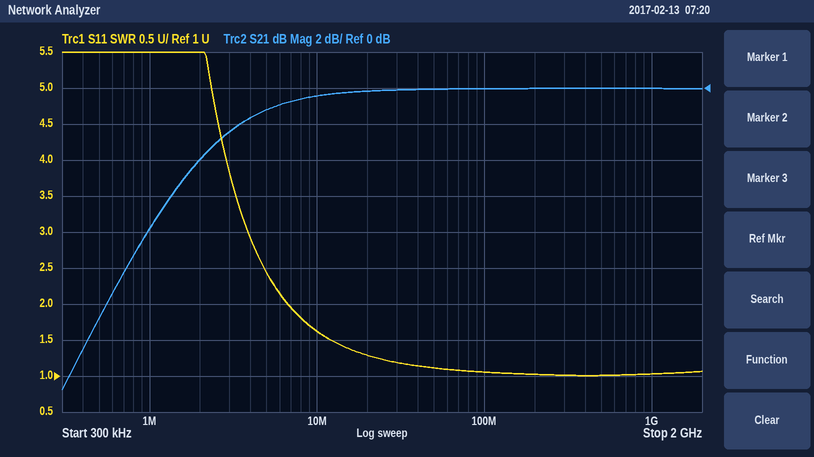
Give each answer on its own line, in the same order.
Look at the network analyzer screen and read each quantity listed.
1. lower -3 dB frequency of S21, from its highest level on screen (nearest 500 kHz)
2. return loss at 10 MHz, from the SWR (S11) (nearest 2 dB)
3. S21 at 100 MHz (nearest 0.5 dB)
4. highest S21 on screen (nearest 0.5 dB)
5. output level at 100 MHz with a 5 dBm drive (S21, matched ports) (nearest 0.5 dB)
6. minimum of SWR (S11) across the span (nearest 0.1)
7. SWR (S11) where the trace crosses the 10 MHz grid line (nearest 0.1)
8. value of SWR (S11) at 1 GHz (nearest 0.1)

2.5 MHz
12 dB
0.0 dB
0.0 dB
5.0 dBm
1.0
1.6
1.0
